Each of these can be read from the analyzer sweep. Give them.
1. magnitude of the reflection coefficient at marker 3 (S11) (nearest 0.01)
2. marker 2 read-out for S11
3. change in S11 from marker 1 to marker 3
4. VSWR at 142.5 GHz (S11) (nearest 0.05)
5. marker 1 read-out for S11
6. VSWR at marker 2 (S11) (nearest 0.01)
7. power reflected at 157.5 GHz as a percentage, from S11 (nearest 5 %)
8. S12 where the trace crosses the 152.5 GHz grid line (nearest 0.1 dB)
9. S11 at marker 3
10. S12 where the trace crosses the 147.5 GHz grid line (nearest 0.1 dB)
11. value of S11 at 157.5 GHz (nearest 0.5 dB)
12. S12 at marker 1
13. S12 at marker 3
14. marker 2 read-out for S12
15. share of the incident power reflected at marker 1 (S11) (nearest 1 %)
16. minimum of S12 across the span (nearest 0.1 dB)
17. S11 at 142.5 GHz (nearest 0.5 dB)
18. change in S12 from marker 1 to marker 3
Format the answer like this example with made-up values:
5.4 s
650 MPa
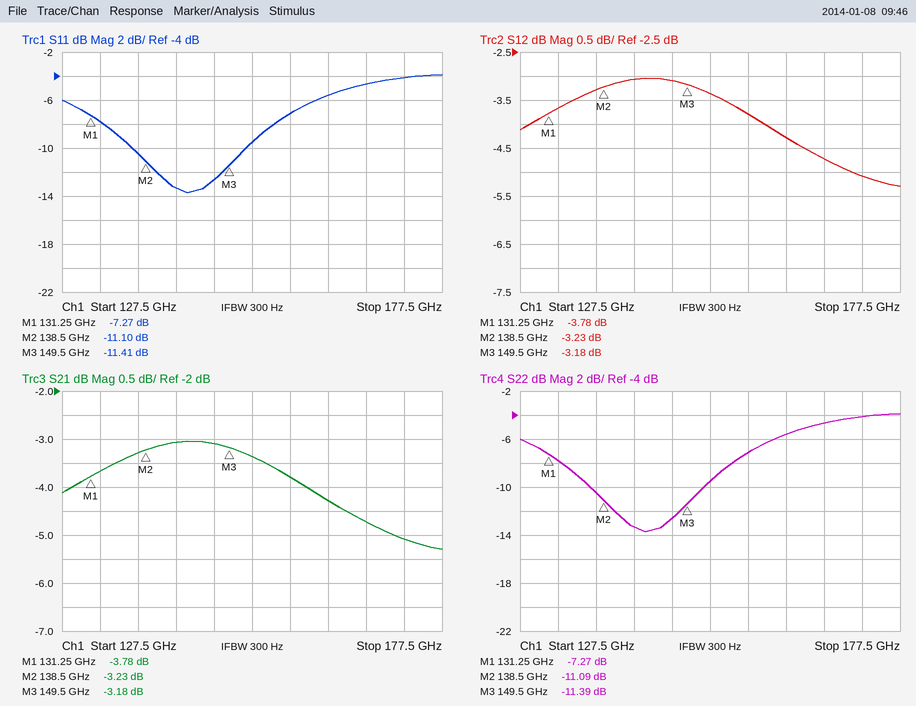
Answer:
0.27
-11.10 dB
-4.14 dB
1.55
-7.27 dB
1.77
20 %
-3.4 dB
-11.41 dB
-3.1 dB
-7.0 dB
-3.78 dB
-3.18 dB
-3.23 dB
19 %
-5.3 dB
-13.5 dB
0.60 dB
